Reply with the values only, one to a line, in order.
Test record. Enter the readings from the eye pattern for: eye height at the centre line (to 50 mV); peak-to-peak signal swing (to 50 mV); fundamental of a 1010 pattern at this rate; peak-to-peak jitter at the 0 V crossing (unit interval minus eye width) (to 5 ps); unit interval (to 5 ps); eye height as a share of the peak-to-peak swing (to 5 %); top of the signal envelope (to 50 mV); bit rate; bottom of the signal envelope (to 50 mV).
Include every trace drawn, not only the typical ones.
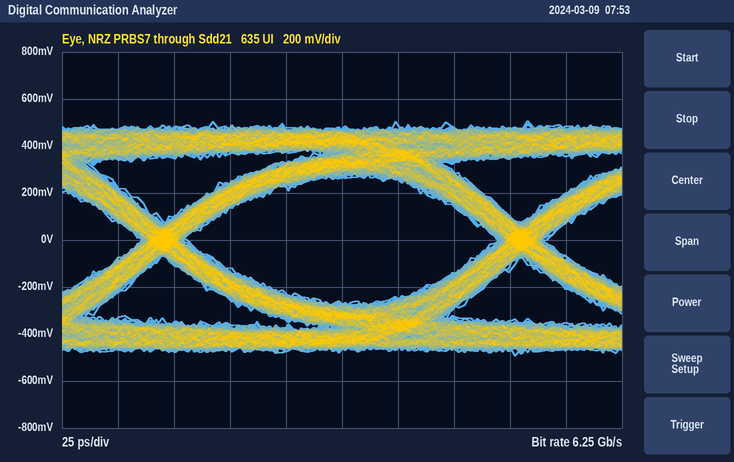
550 mV
1.00 V
3.125 GHz
20 ps
160 ps
55 %
500 mV
6.25 Gb/s
-500 mV
